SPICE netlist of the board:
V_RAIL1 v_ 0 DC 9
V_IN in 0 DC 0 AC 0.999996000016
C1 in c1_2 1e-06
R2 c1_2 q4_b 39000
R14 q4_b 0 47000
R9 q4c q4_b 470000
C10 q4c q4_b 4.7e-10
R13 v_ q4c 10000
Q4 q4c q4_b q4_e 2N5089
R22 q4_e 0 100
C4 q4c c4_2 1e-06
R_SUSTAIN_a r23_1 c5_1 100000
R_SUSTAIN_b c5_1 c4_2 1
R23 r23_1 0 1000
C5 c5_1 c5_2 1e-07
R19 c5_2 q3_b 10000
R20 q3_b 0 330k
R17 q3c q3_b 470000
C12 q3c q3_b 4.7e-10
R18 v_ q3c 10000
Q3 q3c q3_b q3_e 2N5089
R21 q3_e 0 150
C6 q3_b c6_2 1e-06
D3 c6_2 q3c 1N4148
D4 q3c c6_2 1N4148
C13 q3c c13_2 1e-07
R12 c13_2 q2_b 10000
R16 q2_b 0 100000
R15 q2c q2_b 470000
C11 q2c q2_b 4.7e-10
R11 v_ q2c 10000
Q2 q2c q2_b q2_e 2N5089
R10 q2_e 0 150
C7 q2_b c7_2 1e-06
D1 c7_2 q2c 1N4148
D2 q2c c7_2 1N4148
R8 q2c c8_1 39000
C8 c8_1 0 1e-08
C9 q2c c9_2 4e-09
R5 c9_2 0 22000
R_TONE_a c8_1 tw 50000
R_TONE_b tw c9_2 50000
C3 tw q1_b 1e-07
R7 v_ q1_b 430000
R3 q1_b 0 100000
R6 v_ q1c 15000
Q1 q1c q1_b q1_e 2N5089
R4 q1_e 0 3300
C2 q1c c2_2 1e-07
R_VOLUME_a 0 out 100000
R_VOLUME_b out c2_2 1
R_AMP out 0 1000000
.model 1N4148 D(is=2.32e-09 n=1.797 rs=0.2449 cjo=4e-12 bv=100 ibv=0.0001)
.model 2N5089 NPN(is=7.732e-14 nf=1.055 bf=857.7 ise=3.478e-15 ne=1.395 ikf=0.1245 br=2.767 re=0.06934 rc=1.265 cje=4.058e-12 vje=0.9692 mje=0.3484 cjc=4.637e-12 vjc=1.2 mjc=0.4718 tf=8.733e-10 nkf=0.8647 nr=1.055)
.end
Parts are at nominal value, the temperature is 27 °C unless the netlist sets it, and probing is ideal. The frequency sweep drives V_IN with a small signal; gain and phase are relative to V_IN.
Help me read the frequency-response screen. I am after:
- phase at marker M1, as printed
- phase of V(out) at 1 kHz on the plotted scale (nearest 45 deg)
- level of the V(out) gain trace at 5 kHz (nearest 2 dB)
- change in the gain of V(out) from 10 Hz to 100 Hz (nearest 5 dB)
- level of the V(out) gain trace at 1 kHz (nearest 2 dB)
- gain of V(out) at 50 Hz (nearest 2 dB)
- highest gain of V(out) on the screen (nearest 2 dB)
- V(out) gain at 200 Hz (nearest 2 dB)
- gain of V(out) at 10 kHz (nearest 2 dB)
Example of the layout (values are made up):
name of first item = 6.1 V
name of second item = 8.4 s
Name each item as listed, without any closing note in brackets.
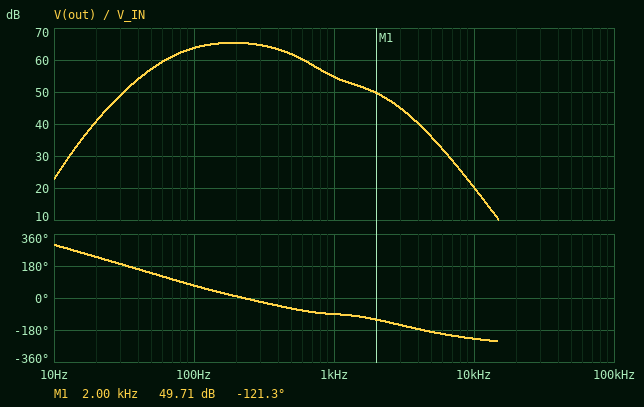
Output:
phase at marker M1, as printed = -121.3 deg
phase of V(out) at 1 kHz on the plotted scale = -90 deg
level of the V(out) gain trace at 5 kHz = 36 dB
change in the gain of V(out) from 10 Hz to 100 Hz = 40 dB
level of the V(out) gain trace at 1 kHz = 54 dB
gain of V(out) at 50 Hz = 58 dB
highest gain of V(out) on the screen = 66 dB
V(out) gain at 200 Hz = 66 dB
gain of V(out) at 10 kHz = 20 dB
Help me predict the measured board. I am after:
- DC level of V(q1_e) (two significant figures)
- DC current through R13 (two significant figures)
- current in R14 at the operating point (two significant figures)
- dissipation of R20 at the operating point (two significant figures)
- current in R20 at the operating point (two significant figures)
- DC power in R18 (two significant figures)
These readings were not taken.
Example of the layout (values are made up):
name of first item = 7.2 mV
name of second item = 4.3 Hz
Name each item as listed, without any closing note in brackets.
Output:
DC level of V(q1_e) = 1.1 V
DC current through R13 = 210 µA
current in R14 at the operating point = 13 µA
dissipation of R20 at the operating point = 1.6 µW
current in R20 at the operating point = 2.2 µA
DC power in R18 = 4.6 mW
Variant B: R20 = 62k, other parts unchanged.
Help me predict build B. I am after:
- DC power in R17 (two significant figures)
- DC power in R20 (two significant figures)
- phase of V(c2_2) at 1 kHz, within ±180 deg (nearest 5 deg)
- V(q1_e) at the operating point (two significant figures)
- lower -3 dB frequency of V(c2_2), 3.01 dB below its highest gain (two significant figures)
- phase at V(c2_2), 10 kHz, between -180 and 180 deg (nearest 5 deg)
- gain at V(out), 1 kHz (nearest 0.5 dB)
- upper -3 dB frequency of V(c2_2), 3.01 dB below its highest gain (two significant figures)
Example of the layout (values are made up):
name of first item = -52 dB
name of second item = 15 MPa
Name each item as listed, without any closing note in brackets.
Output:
DC power in R17 = 56 µW
DC power in R20 = 6.8 µW
phase of V(c2_2) at 1 kHz, within ±180 deg = -85 deg
V(q1_e) at the operating point = 1.1 V
lower -3 dB frequency of V(c2_2), 3.01 dB below its highest gain = 80 Hz
phase at V(c2_2), 10 kHz, between -180 and 180 deg = 135 deg
gain at V(out), 1 kHz = 53.5 dB
upper -3 dB frequency of V(c2_2), 3.01 dB below its highest gain = 470 Hz
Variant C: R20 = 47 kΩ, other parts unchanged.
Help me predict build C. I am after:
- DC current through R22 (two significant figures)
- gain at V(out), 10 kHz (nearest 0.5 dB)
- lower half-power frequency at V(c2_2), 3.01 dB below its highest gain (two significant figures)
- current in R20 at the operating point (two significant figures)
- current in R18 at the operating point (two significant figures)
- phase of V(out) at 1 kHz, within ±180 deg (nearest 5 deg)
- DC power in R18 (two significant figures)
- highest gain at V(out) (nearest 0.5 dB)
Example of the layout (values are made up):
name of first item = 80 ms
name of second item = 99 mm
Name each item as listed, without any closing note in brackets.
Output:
DC current through R22 = 200 µA
gain at V(out), 10 kHz = 19.5 dB
lower half-power frequency at V(c2_2), 3.01 dB below its highest gain = 78 Hz
current in R20 at the operating point = 13 µA
current in R18 at the operating point = 210 µA
phase of V(out) at 1 kHz, within ±180 deg = -85 deg
DC power in R18 = 420 µW
highest gain at V(out) = 62.5 dB
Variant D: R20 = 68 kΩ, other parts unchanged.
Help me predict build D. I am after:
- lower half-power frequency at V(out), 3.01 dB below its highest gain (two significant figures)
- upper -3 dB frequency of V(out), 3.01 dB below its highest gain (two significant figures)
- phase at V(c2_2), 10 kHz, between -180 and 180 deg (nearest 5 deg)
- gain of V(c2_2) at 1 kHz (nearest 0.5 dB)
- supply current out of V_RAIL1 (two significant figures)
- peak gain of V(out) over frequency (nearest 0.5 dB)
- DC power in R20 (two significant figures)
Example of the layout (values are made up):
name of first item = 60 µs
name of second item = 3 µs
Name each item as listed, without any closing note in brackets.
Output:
lower half-power frequency at V(out), 3.01 dB below its highest gain = 80 Hz
upper -3 dB frequency of V(out), 3.01 dB below its highest gain = 470 Hz
phase at V(c2_2), 10 kHz, between -180 and 180 deg = 135 deg
gain of V(c2_2) at 1 kHz = 53.5 dB
supply current out of V_RAIL1 = 1.4 mA
peak gain of V(out) over frequency = 64.0 dB
DC power in R20 = 6.4 µW
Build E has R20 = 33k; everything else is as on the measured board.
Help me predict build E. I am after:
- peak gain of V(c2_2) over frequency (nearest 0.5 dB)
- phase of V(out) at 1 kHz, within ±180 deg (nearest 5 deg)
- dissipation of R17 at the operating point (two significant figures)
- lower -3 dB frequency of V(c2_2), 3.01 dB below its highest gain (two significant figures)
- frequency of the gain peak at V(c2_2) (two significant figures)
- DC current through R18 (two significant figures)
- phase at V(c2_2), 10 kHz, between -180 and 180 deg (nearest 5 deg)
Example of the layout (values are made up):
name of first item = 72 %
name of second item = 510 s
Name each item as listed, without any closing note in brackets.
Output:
peak gain of V(c2_2) over frequency = 55.0 dB
phase of V(out) at 1 kHz, within ±180 deg = -75 deg
dissipation of R17 at the operating point = 130 µW
lower -3 dB frequency of V(c2_2), 3.01 dB below its highest gain = 70 Hz
frequency of the gain peak at V(c2_2) = 180 Hz
DC current through R18 = 55 µA
phase at V(c2_2), 10 kHz, between -180 and 180 deg = 150 deg
